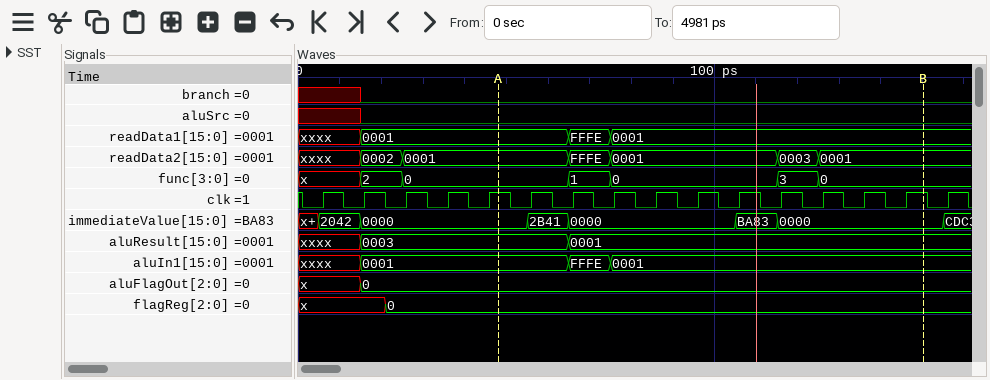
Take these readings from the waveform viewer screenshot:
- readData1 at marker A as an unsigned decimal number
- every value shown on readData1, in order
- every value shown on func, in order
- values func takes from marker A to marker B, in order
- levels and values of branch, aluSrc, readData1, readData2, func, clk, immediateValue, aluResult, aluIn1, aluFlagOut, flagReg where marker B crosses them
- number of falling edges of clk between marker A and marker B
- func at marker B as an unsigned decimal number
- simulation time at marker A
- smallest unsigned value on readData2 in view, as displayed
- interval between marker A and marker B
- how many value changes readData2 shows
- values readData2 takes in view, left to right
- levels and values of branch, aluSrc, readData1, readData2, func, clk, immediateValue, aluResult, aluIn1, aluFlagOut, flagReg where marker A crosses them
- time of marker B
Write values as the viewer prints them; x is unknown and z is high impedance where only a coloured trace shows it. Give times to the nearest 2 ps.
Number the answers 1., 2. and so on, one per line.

1. 1
2. xxxx, 0001, FFFE, 0001
3. x, 2, 0, 1, 0, 3, 0
4. 0, 1, 0, 3, 0
5. branch=0, aluSrc=0, readData1=0001, readData2=0001, func=0, clk=1, immediateValue=0000, aluResult=0001, aluIn1=0001, aluFlagOut=0, flagReg=0
6. 10
7. 0
8. 48 ps
9. 0001
10. 102 ps
11. 6
12. xxxx, 0002, 0001, FFFE, 0001, 0003, 0001
13. branch=0, aluSrc=0, readData1=0001, readData2=0001, func=0, clk=1, immediateValue=0000, aluResult=0003, aluIn1=0001, aluFlagOut=0, flagReg=0
14. 150 ps
